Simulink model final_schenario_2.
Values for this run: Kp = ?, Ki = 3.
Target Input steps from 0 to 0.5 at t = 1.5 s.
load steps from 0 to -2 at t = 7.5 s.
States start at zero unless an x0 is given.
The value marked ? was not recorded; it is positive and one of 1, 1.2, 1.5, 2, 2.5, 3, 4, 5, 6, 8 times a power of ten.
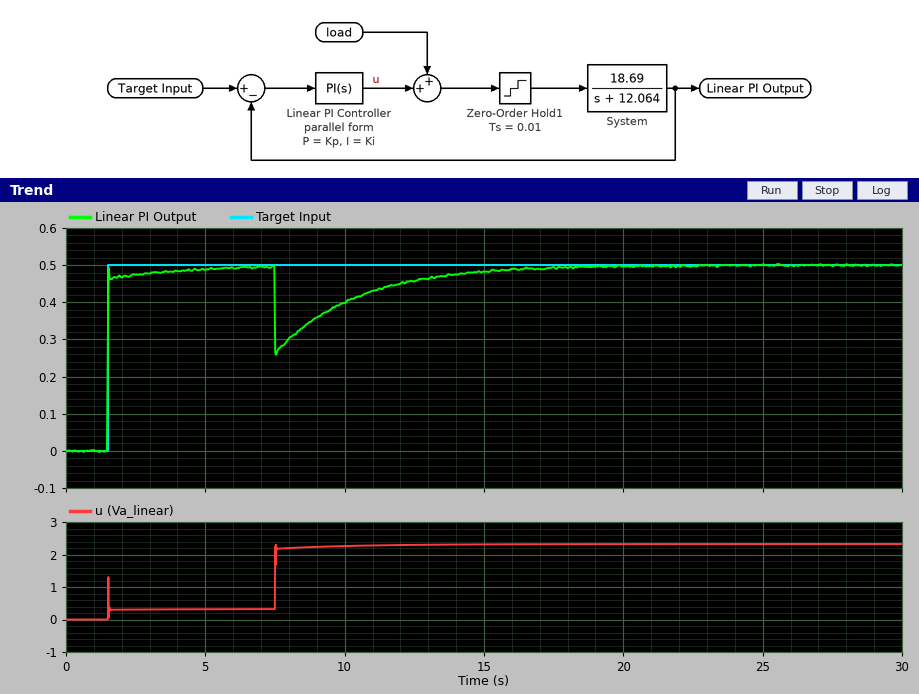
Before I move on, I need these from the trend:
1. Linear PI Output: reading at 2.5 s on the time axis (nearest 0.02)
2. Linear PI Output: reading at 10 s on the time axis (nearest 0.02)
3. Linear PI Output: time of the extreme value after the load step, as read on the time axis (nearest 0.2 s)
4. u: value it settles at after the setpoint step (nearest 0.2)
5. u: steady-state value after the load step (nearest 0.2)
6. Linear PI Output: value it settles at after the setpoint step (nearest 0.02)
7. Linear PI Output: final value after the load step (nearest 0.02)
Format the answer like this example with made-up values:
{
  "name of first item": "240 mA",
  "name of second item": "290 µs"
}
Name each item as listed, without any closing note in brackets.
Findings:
{
  "Linear PI Output: reading at 2.5 s on the time axis": "0.48",
  "Linear PI Output: reading at 10 s on the time axis": "0.40",
  "Linear PI Output: time of the extreme value after the load step, as read on the time axis": "7.6 s",
  "u: value it settles at after the setpoint step": "0.4",
  "u: steady-state value after the load step": "2.4",
  "Linear PI Output: value it settles at after the setpoint step": "0.50",
  "Linear PI Output: final value after the load step": "0.50"
}
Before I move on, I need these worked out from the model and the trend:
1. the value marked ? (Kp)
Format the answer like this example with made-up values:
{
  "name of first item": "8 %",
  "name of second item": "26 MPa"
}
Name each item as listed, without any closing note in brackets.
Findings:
{
  "the value marked ?": "8"
}
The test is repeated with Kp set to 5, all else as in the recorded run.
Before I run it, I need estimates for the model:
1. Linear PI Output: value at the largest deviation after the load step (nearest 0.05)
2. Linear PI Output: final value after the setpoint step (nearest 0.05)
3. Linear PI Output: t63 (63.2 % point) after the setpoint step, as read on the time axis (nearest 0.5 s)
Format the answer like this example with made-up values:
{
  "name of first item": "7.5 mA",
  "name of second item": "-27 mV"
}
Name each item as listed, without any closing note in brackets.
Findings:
{
  "Linear PI Output: value at the largest deviation after the load step": "0.15",
  "Linear PI Output: final value after the setpoint step": "0.50",
  "Linear PI Output: t63 (63.2 % point) after the setpoint step, as read on the time axis": "1.5 s"
}
